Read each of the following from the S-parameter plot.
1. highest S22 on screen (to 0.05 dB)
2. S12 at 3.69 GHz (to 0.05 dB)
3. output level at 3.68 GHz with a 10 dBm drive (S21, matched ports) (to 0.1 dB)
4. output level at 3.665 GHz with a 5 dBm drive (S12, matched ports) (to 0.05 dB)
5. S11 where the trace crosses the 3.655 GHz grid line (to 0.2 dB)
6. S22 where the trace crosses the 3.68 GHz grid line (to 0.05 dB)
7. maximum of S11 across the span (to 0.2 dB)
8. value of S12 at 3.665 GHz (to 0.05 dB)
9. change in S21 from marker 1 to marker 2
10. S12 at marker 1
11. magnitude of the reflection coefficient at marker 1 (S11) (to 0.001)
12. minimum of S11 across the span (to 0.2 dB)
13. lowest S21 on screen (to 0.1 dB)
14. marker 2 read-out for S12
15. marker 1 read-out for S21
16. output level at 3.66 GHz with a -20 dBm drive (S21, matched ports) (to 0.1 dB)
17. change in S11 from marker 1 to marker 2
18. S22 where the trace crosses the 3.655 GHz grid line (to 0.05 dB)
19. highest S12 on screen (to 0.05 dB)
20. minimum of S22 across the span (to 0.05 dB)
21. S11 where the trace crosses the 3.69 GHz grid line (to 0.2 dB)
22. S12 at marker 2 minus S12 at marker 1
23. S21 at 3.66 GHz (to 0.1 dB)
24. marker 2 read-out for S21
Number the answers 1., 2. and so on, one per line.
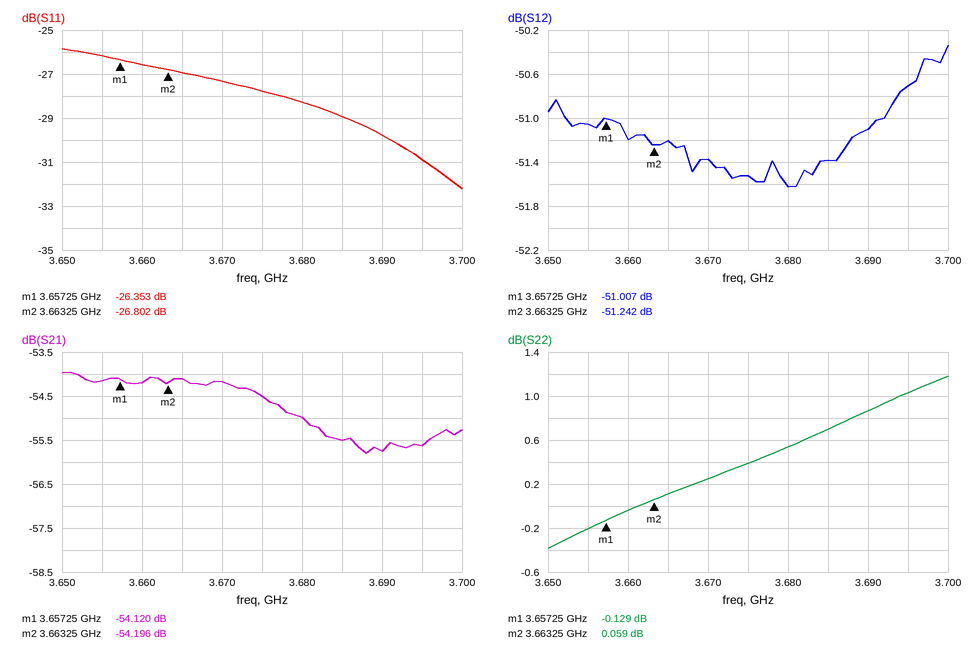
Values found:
1. 1.20 dB
2. -51.10 dB
3. -45.0 dBm
4. -46.20 dBm
5. -26.2 dB
6. 0.55 dB
7. -25.8 dB
8. -51.20 dB
9. -0.076 dB
10. -51.007 dB
11. 0.048
12. -32.2 dB
13. -55.8 dB
14. -51.242 dB
15. -54.120 dB
16. -74.2 dBm
17. -0.449 dB
18. -0.20 dB
19. -50.35 dB
20. -0.40 dB
21. -29.8 dB
22. -0.235 dB
23. -54.2 dB
24. -54.196 dB
